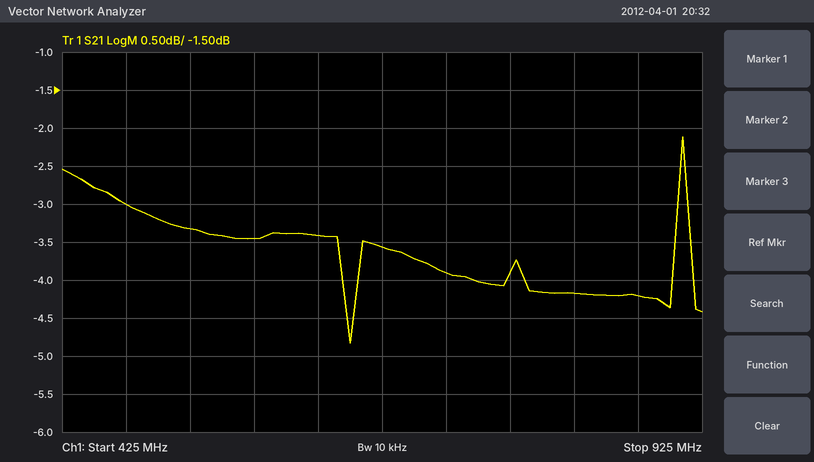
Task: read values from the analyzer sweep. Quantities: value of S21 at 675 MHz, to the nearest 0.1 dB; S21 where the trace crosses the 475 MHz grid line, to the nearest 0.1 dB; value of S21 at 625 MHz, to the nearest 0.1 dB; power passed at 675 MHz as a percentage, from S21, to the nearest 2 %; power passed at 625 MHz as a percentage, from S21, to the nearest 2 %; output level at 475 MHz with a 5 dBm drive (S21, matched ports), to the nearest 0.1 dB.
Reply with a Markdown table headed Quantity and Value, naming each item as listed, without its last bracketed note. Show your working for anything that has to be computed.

| Quantity | Value |
|---|---|
| value of S21 at 675 MHz, to the nearest 0.1 dB | -3.6 dB |
| S21 where the trace crosses the 475 MHz grid line, to the nearest 0.1 dB | -3.0 dB |
| value of S21 at 625 MHz, to the nearest 0.1 dB | -3.4 dB |
| power passed at 675 MHz as a percentage, from S21, to the nearest 2 % | 10^(-3.6/10) ≈ 44 % |
| power passed at 625 MHz as a percentage, from S21, to the nearest 2 % | 10^(-3.4/10) ≈ 46 % |
| output level at 475 MHz with a 5 dBm drive (S21, matched ports), to the nearest 0.1 dB | 5 dBm + (-3.0 dB) = 2.0 dBm |
